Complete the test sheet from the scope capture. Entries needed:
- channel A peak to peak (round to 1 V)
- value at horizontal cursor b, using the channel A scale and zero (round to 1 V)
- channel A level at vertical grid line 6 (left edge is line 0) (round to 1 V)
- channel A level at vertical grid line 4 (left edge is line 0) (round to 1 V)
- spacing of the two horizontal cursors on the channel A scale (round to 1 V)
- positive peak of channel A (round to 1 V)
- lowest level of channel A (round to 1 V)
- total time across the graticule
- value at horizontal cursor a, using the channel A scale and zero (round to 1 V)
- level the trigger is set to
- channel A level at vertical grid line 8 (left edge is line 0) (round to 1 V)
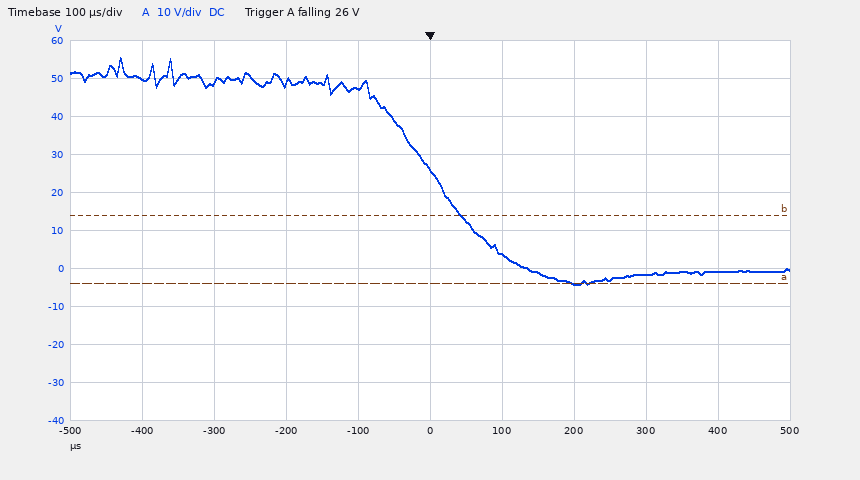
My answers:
60 V
14 V
4 V
47 V
18 V
56 V
-4 V
1 ms
-4 V
26 V
-2 V
